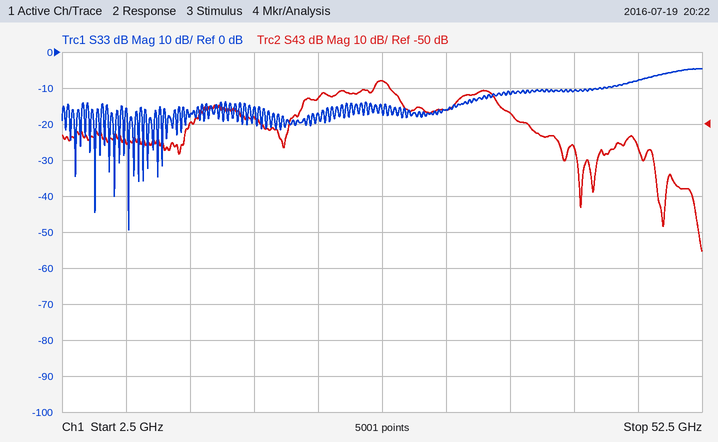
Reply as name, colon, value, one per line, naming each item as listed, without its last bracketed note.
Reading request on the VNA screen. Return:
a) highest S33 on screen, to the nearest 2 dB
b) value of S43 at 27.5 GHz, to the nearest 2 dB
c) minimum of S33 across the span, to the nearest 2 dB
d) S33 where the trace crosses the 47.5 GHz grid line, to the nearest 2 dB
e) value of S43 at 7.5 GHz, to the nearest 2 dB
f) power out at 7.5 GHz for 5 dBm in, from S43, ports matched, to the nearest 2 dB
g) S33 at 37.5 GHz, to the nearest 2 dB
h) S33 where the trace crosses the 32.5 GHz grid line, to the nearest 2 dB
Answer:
highest S33 on screen, to the nearest 2 dB: -4 dB
value of S43 at 27.5 GHz, to the nearest 2 dB: -38 dB
minimum of S33 across the span, to the nearest 2 dB: -50 dB
S33 where the trace crosses the 47.5 GHz grid line, to the nearest 2 dB: -8 dB
value of S43 at 7.5 GHz, to the nearest 2 dB: -56 dB
power out at 7.5 GHz for 5 dBm in, from S43, ports matched, to the nearest 2 dB: -50 dBm
S33 at 37.5 GHz, to the nearest 2 dB: -12 dB
S33 where the trace crosses the 32.5 GHz grid line, to the nearest 2 dB: -16 dB
